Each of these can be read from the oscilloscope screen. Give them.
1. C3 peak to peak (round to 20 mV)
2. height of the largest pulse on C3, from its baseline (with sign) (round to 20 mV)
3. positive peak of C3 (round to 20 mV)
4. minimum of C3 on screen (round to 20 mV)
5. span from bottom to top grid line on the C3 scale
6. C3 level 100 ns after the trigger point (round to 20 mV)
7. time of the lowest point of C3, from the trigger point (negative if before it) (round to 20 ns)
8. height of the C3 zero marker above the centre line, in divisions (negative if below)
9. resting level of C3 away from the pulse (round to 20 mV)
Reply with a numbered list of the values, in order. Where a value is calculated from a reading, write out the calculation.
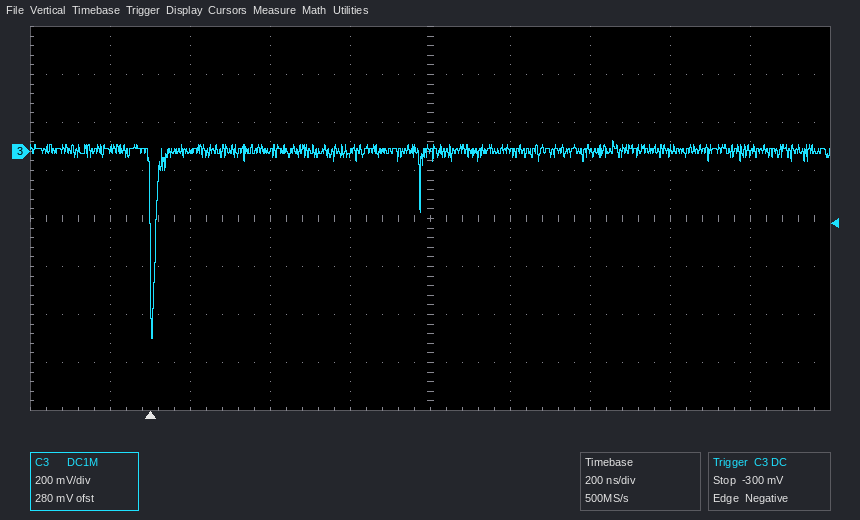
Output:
1. 40 mV − (-780 mV) = 820 mV
2. -780 mV − (0 mV) = -780 mV
3. 40 mV
4. -780 mV
5. 1.6 V
6. 0 mV
7. 0 ns
8. +1.4 div
9. 0 mV
